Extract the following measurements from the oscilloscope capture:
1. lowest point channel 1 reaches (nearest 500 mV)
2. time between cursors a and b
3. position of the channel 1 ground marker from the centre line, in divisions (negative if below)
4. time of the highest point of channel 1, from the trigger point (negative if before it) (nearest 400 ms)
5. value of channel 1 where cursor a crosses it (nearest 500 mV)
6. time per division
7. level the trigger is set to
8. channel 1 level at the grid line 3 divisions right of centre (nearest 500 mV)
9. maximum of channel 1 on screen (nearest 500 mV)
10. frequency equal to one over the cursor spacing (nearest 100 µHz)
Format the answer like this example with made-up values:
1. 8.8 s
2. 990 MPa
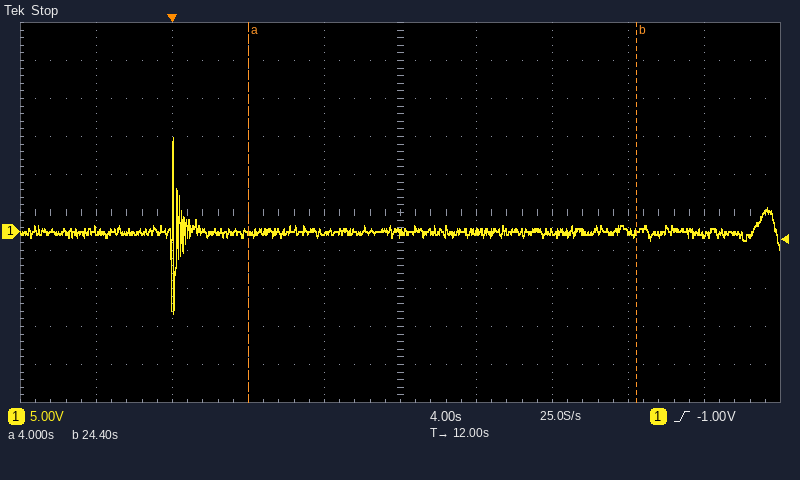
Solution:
1. -11.0 V
2. 20.4 s
3. -0.5 div
4. 0.0 s
5. 0.0 V
6. 4 s
7. -1.00 V
8. 0.0 V
9. 12.5 V
10. 49.0 mHz
